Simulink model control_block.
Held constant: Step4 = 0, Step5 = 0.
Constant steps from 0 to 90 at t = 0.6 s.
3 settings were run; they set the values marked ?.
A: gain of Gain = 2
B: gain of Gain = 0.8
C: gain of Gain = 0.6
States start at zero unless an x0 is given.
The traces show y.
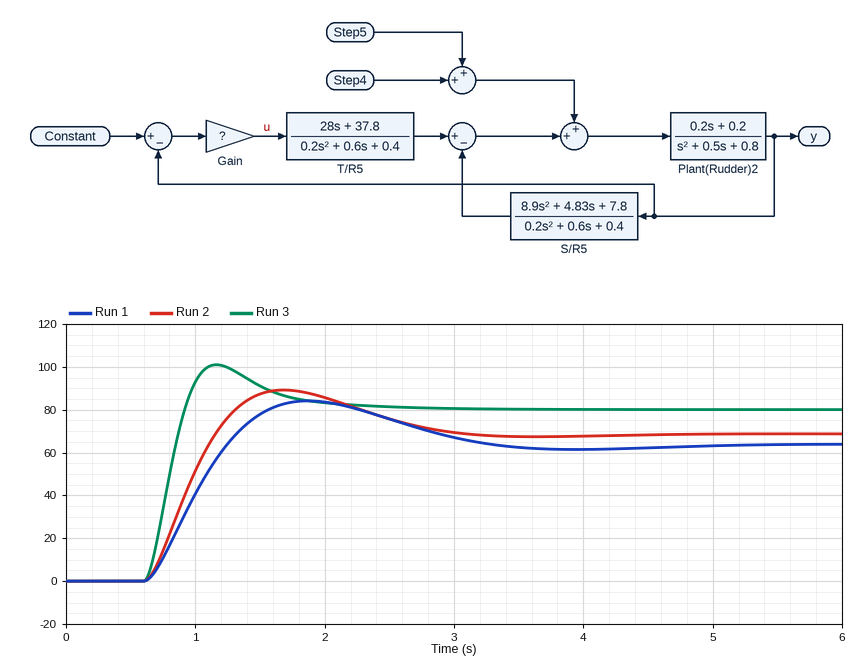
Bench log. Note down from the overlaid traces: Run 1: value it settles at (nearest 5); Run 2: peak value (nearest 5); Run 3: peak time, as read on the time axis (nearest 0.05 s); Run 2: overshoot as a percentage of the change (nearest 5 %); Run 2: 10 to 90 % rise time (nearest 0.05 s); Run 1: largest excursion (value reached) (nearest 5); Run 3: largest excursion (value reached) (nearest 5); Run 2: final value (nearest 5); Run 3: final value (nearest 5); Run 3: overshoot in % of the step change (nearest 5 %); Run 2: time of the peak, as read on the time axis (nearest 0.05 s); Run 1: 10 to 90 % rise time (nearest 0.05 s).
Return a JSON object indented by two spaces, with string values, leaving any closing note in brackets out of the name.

{
  "Run 1: value it settles at": "65",
  "Run 2: peak value": "90",
  "Run 3: peak time, as read on the time axis": "1.15 s",
  "Run 2: overshoot as a percentage of the change": "30 %",
  "Run 2: 10 to 90 % rise time": "0.40 s",
  "Run 1: largest excursion (value reached)": "85",
  "Run 3: largest excursion (value reached)": "100",
  "Run 2: final value": "70",
  "Run 3: final value": "80",
  "Run 3: overshoot in % of the step change": "25 %",
  "Run 2: time of the peak, as read on the time axis": "1.70 s",
  "Run 1: 10 to 90 % rise time": "0.45 s"
}
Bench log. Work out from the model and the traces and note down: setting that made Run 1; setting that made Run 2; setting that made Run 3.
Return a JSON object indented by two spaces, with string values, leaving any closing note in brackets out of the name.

{
  "setting that made Run 1": "C",
  "setting that made Run 2": "B",
  "setting that made Run 3": "A"
}
